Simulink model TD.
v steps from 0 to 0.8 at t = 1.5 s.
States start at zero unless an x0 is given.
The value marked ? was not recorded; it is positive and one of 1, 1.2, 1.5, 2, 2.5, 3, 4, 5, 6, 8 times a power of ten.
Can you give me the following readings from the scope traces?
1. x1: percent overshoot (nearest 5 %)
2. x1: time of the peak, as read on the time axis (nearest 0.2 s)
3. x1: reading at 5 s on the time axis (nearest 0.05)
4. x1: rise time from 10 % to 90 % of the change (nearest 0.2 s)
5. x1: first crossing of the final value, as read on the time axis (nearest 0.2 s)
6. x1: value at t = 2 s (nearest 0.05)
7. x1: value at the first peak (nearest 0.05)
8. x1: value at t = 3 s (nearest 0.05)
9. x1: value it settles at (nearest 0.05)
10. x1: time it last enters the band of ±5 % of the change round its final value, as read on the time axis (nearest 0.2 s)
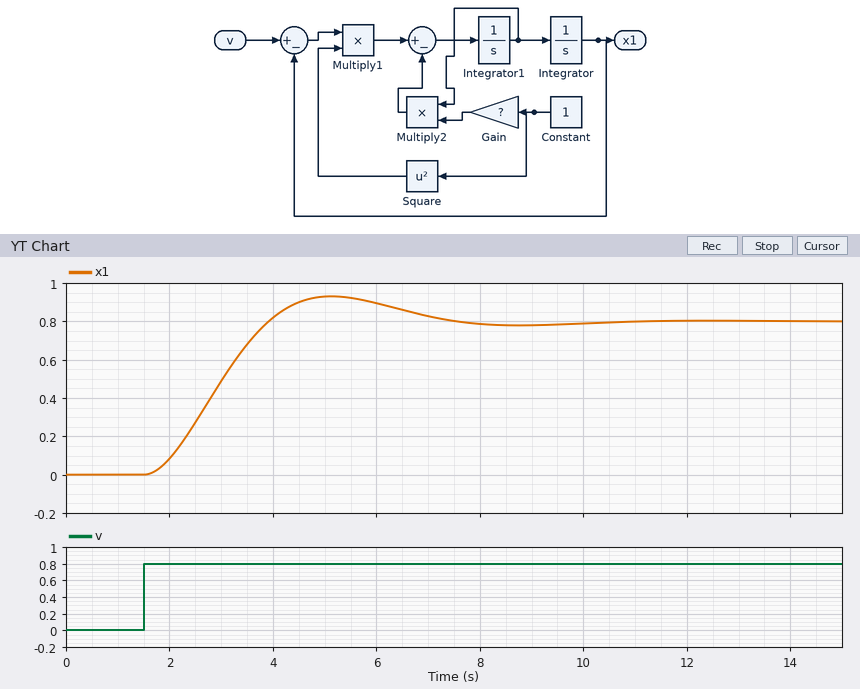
15 %
5.2 s
0.95
1.6 s
4.0 s
0.10
0.95
0.50
0.80
6.8 s
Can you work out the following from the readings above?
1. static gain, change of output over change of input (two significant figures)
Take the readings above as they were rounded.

1.0
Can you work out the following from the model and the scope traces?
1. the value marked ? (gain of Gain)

1
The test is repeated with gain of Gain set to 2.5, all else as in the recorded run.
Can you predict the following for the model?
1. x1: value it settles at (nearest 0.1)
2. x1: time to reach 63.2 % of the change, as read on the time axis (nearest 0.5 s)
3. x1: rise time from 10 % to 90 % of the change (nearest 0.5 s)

0.8
4.0 s
4.5 s
